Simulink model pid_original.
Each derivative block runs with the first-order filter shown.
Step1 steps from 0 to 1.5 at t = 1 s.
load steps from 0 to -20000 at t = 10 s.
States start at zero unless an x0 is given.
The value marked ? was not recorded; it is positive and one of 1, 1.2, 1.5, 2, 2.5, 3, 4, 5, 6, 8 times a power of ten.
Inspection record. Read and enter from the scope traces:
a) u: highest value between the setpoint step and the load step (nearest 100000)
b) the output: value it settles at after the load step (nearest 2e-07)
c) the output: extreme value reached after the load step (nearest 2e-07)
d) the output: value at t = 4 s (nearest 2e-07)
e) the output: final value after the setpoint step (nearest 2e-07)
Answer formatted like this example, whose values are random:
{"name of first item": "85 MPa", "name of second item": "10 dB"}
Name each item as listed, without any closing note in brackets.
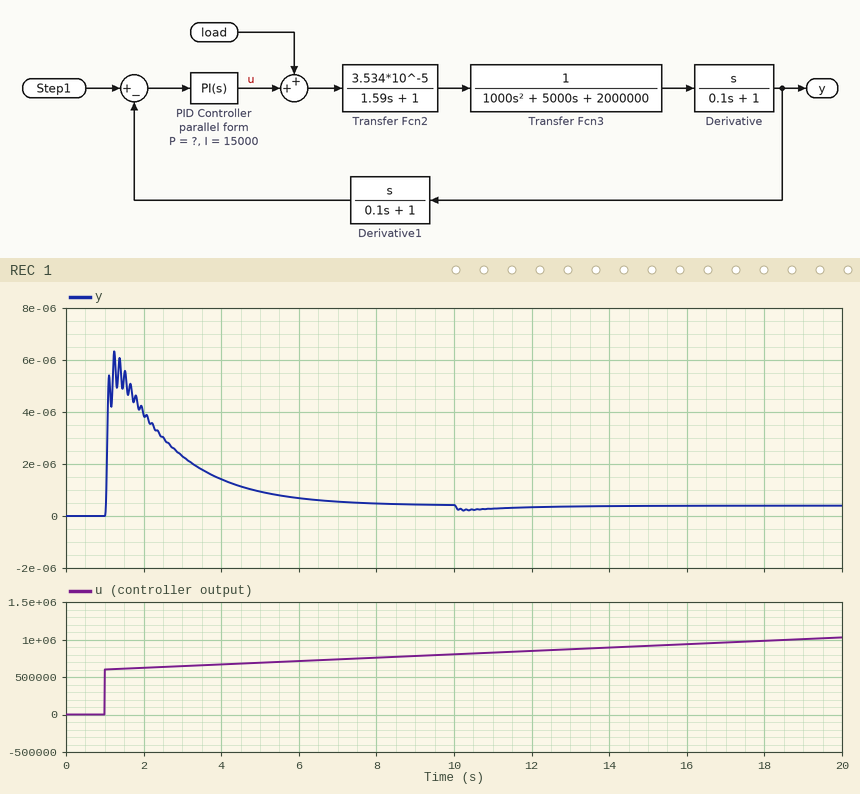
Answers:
{"u: highest value between the setpoint step and the load step": "800000", "the output: value it settles at after the load step": "0.0000004", "the output: extreme value reached after the load step": "0.0000002", "the output: value at t = 4 s": "0.0000014", "the output: final value after the setpoint step": "0.0000004"}
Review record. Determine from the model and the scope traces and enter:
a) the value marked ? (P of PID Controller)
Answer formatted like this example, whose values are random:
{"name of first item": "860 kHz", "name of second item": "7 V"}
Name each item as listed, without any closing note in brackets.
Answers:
{"the value marked ?": "400000"}
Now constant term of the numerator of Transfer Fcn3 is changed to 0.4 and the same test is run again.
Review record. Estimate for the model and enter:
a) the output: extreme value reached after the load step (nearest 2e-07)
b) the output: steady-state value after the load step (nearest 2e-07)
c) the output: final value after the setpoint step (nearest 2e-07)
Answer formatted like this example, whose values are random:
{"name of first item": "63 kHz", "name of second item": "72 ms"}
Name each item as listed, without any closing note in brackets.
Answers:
{"the output: extreme value reached after the load step": "0.0000000", "the output: steady-state value after the load step": "0.0000002", "the output: final value after the setpoint step": "0.0000002"}
